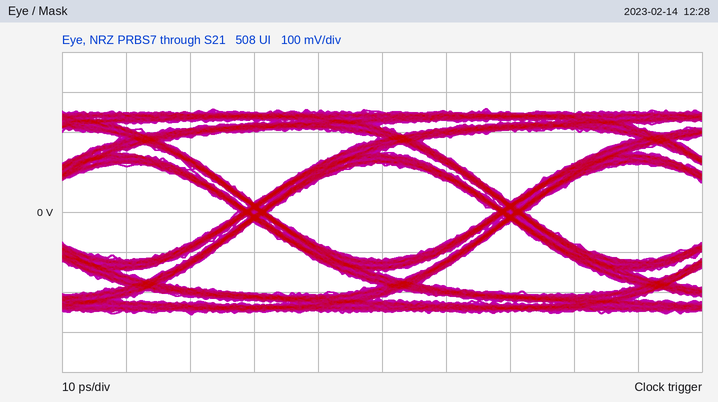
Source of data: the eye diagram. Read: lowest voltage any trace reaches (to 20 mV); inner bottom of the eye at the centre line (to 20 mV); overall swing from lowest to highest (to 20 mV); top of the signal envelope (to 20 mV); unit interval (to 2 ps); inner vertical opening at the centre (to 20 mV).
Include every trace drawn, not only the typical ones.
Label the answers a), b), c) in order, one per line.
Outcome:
a) -260 mV
b) -120 mV
c) 520 mV
d) 260 mV
e) 40 ps
f) 240 mV
